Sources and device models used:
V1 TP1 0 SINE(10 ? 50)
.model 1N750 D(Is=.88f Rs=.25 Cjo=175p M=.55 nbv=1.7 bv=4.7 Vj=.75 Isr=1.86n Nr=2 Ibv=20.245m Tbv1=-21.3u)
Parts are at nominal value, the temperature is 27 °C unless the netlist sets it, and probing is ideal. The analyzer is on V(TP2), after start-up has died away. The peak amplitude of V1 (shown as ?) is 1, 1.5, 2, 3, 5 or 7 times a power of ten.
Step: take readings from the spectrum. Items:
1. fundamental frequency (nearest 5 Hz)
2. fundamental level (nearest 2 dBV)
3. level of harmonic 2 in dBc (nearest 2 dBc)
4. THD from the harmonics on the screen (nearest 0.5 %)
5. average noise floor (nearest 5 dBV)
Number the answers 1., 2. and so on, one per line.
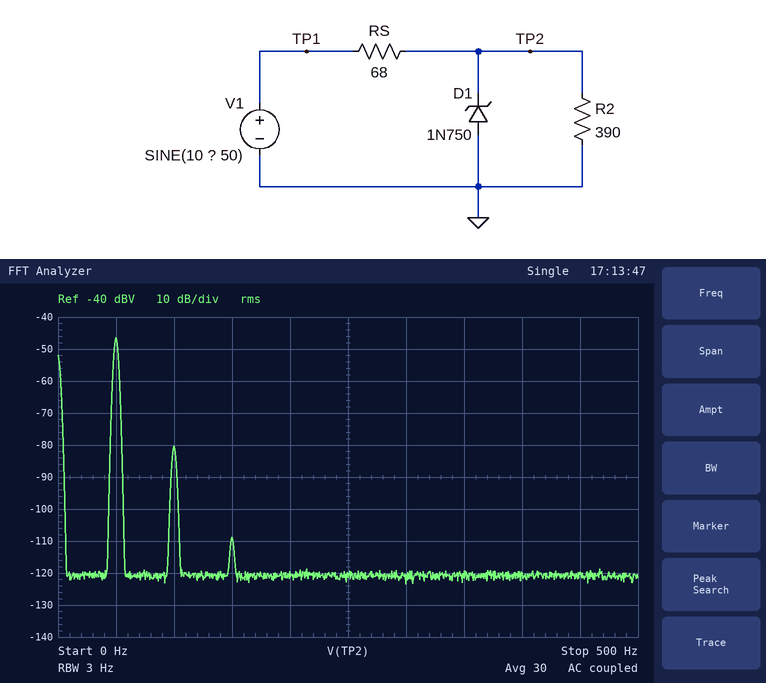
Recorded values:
1. 50 Hz
2. -46 dBV
3. -34 dBc
4. 2.0 %
5. -120 dBV
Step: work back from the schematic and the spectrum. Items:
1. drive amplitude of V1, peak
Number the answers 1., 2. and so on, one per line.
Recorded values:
1. 500 mV
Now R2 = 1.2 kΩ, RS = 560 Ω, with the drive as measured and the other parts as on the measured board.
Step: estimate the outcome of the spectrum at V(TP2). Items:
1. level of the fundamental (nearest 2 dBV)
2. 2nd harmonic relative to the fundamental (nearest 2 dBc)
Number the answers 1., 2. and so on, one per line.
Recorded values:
1. -46 dBV
2. -28 dBc
